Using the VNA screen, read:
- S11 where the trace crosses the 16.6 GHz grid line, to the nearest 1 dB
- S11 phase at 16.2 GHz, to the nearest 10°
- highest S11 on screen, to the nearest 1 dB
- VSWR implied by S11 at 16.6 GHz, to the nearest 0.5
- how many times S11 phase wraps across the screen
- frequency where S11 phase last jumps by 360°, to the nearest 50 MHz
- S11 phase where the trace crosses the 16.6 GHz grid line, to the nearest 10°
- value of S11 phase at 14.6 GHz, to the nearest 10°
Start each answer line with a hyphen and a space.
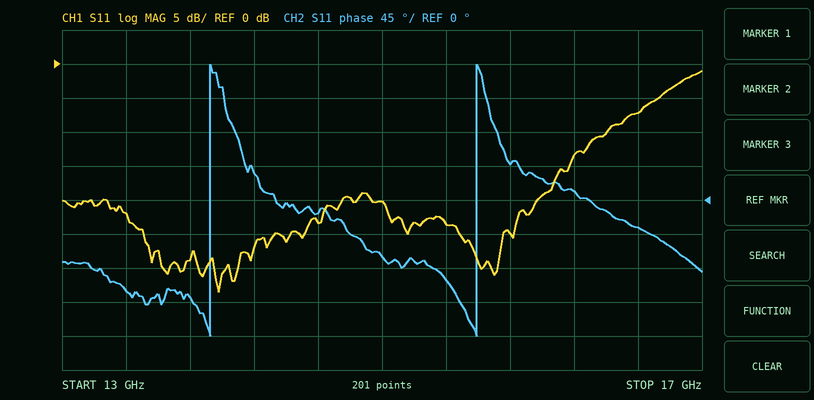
- -7 dB
- 10°
- -1 dB
- 2.5
- 2
- 15.60 GHz
- -40°
- -20°
